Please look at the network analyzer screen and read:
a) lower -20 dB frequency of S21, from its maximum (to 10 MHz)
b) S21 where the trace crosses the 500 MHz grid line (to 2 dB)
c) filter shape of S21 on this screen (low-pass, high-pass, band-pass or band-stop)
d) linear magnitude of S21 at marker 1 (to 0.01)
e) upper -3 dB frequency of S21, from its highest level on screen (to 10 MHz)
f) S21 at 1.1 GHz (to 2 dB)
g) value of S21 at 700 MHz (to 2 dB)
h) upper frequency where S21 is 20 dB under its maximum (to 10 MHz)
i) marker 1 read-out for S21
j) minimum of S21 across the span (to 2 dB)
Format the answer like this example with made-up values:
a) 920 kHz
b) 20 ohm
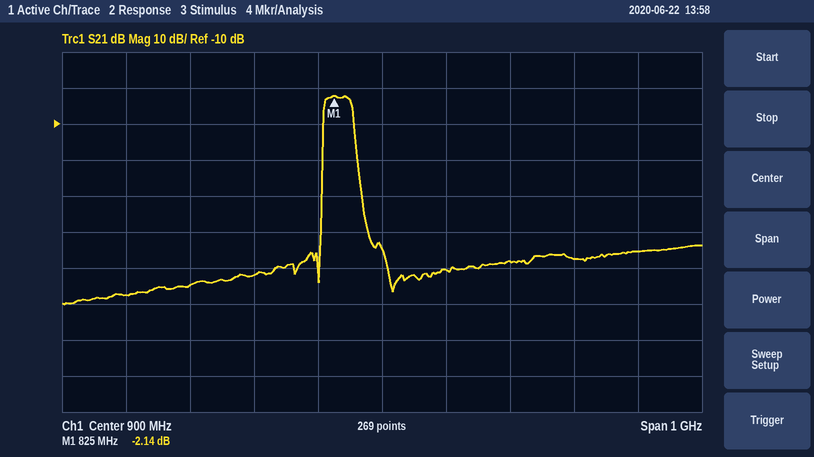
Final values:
a) 810 MHz
b) -58 dB
c) band-pass
d) 0.78
e) 850 MHz
f) -48 dB
g) -52 dB
h) 860 MHz
i) -2.14 dB
j) -60 dB
